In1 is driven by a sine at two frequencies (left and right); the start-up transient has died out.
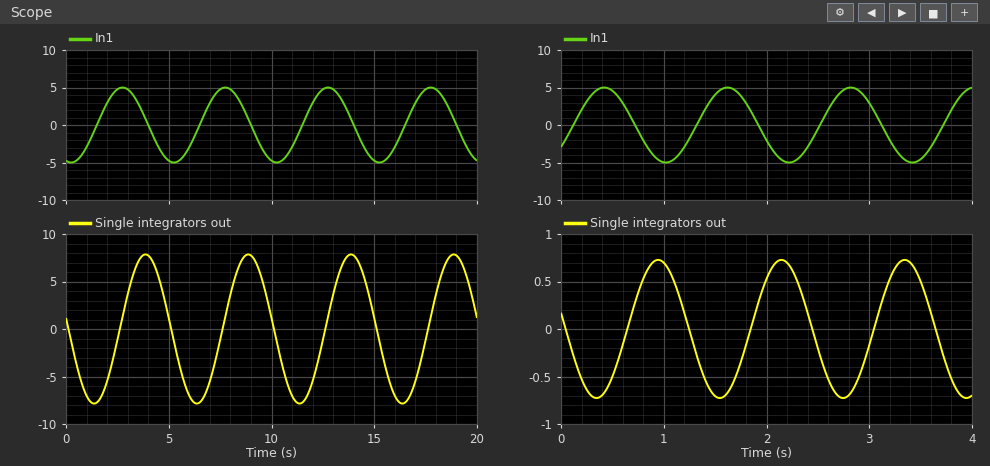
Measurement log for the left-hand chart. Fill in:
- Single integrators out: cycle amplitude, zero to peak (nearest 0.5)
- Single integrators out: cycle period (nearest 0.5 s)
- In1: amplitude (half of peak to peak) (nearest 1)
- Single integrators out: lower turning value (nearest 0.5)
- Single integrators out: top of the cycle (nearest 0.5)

8.0
5.0 s
5
-8.0
8.0
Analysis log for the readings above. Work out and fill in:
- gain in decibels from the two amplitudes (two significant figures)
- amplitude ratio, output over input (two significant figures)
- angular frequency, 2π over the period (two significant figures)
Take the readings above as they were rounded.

4.1 dB
1.6
1.3 rad/s
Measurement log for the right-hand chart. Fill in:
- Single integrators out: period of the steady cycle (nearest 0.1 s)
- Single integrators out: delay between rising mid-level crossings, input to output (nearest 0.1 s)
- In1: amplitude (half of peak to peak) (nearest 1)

1.2 s
0.5 s
5
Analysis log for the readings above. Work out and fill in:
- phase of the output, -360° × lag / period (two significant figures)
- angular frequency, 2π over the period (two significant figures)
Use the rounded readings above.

-150°
5.2 rad/s
